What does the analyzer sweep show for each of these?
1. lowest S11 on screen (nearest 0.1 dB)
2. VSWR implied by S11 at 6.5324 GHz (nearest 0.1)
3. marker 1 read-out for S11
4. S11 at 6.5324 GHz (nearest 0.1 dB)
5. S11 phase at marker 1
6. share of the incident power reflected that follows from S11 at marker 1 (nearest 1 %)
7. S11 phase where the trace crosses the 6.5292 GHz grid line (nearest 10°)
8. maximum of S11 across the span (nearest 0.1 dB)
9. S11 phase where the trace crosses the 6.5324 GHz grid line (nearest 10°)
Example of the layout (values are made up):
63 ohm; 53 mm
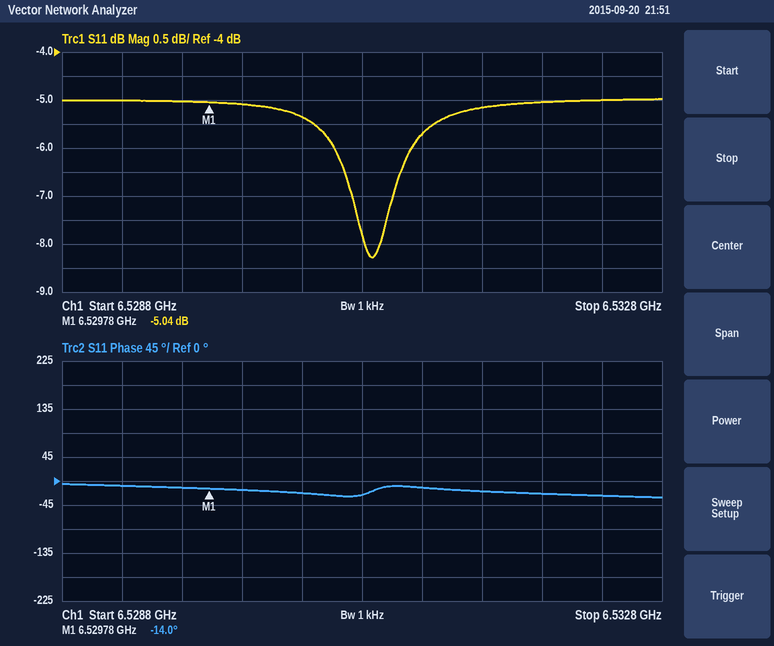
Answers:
-8.3 dB; 3.6; -5.04 dB; -5.0 dB; -14.0°; 31 %; -10°; -5.0 dB; -30°
